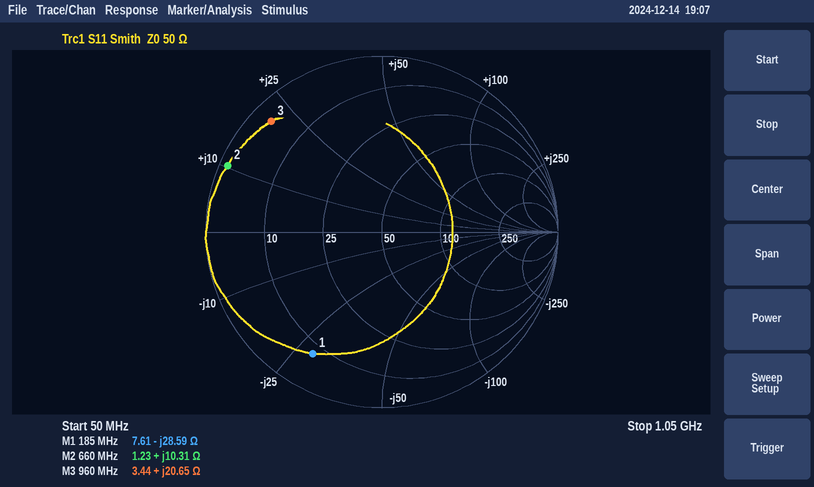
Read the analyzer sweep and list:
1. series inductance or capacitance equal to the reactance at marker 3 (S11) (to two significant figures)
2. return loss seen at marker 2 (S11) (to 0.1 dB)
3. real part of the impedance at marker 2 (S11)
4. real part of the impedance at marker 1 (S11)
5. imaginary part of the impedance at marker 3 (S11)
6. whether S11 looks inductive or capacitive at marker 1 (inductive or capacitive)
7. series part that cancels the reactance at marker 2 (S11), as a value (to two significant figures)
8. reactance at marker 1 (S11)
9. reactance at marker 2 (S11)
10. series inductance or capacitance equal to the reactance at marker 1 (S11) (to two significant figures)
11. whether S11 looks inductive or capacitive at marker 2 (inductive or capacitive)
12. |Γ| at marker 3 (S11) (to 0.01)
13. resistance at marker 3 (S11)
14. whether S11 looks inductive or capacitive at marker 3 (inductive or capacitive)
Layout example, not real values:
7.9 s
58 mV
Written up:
3.4 nH
0.4 dB
1.23 Ω
7.61 Ω
+20.65 Ω
capacitive
23 pF
-28.59 Ω
+10.31 Ω
30 pF
inductive
0.89
3.44 Ω
inductive
